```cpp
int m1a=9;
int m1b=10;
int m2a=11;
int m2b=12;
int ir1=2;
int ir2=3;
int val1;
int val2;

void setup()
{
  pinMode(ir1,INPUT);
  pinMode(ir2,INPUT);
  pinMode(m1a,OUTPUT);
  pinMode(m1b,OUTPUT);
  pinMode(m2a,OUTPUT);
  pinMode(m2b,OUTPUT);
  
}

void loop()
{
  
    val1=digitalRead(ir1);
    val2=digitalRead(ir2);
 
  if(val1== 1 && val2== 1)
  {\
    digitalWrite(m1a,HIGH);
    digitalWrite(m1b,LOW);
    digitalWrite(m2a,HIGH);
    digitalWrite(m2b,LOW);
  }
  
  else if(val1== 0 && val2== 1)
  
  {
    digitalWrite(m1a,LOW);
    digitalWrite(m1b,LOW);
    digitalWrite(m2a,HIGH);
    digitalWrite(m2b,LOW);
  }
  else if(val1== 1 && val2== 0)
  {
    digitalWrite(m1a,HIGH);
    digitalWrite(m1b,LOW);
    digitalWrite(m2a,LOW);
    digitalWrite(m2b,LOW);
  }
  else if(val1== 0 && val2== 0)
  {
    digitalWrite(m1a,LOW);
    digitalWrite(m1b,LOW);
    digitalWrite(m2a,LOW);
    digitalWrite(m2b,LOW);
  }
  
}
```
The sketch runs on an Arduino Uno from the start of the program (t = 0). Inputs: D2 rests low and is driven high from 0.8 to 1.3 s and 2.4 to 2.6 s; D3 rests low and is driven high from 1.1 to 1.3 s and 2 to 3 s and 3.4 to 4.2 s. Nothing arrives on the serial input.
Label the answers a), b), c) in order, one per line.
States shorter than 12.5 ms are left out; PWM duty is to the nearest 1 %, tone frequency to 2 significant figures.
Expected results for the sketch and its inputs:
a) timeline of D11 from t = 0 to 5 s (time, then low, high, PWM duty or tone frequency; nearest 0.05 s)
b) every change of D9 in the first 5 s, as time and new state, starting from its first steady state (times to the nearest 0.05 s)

a) 0 s low; 1.1 s high; 1.3 s low; 2 s high; 3 s low; 3.4 s high; 4.2 s low
b) 0 s low; 0.8 s high; 1.3 s low; 2.4 s high; 2.6 s low
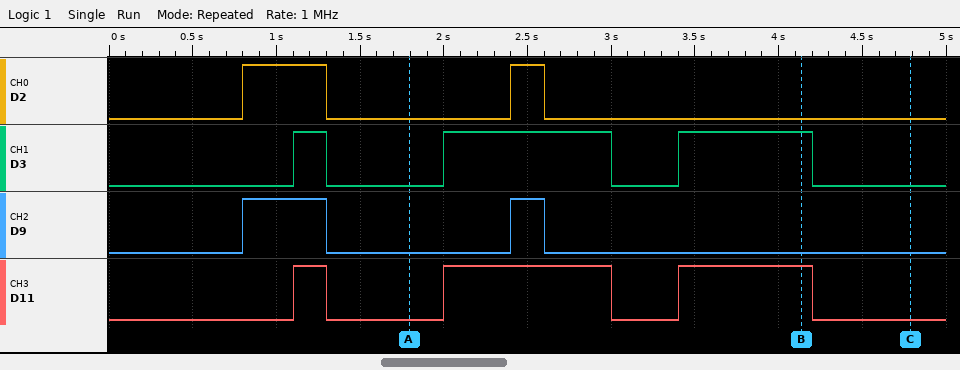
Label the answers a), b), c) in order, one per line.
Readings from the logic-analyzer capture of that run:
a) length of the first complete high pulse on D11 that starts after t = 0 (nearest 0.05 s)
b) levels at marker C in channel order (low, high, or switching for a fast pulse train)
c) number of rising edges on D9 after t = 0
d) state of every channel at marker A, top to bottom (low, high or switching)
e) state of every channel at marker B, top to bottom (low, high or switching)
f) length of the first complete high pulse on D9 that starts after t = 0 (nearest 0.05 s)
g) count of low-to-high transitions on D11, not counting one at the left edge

a) 0.20 s
b) D2 low, D3 low, D9 low, D11 low
c) 2
d) D2 low, D3 low, D9 low, D11 low
e) D2 low, D3 high, D9 low, D11 high
f) 0.50 s
g) 3
